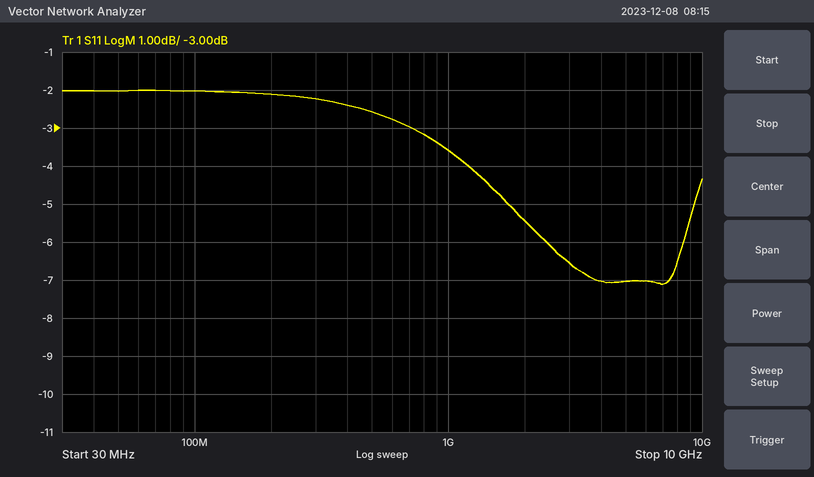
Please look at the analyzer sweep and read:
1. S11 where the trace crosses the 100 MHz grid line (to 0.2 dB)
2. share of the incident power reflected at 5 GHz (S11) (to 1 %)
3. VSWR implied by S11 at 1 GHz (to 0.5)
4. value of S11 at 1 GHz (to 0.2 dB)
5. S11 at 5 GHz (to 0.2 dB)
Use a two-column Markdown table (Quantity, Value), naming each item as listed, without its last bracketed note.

| Quantity | Value |
|---|---|
| S11 where the trace crosses the 100 MHz grid line | -2.0 dB |
| share of the incident power reflected at 5 GHz (S11) | 20 % |
| VSWR implied by S11 at 1 GHz | 5.0 |
| value of S11 at 1 GHz | -3.6 dB |
| S11 at 5 GHz | -7.0 dB |
